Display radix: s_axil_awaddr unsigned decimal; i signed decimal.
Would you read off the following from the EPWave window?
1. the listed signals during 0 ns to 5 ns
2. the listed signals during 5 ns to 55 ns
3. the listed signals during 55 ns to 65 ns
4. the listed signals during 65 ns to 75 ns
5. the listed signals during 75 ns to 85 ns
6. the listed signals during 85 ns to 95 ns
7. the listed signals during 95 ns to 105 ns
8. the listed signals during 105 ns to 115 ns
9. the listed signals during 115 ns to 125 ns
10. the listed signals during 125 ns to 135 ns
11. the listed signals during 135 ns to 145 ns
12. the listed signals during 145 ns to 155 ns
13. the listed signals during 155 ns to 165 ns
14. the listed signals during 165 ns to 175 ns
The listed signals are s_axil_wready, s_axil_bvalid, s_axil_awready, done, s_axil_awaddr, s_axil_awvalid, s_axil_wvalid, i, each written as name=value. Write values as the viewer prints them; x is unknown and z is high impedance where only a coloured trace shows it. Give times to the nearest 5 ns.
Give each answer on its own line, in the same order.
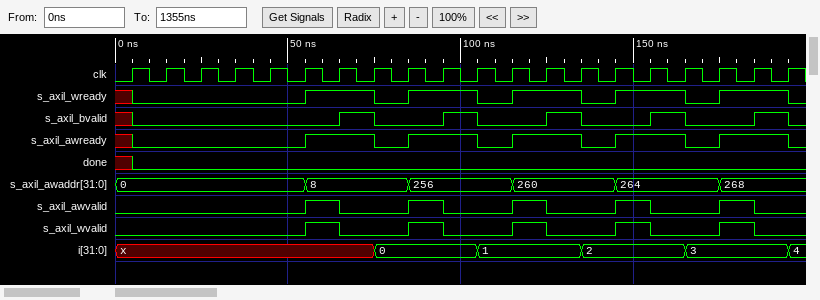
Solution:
s_axil_wready=x, s_axil_bvalid=x, s_axil_awready=x, done=x, s_axil_awaddr=0, s_axil_awvalid=0, s_axil_wvalid=0, i=x
s_axil_wready=0, s_axil_bvalid=0, s_axil_awready=0, done=0, s_axil_awaddr=0, s_axil_awvalid=0, s_axil_wvalid=0, i=x
s_axil_wready=1, s_axil_bvalid=0, s_axil_awready=1, done=0, s_axil_awaddr=8, s_axil_awvalid=1, s_axil_wvalid=1, i=x
s_axil_wready=1, s_axil_bvalid=1, s_axil_awready=1, done=0, s_axil_awaddr=8, s_axil_awvalid=0, s_axil_wvalid=0, i=x
s_axil_wready=0, s_axil_bvalid=0, s_axil_awready=0, done=0, s_axil_awaddr=8, s_axil_awvalid=0, s_axil_wvalid=0, i=0
s_axil_wready=1, s_axil_bvalid=0, s_axil_awready=1, done=0, s_axil_awaddr=256, s_axil_awvalid=1, s_axil_wvalid=1, i=0
s_axil_wready=1, s_axil_bvalid=1, s_axil_awready=1, done=0, s_axil_awaddr=256, s_axil_awvalid=0, s_axil_wvalid=0, i=0
s_axil_wready=0, s_axil_bvalid=0, s_axil_awready=0, done=0, s_axil_awaddr=256, s_axil_awvalid=0, s_axil_wvalid=0, i=1
s_axil_wready=1, s_axil_bvalid=0, s_axil_awready=1, done=0, s_axil_awaddr=260, s_axil_awvalid=1, s_axil_wvalid=1, i=1
s_axil_wready=1, s_axil_bvalid=1, s_axil_awready=1, done=0, s_axil_awaddr=260, s_axil_awvalid=0, s_axil_wvalid=0, i=1
s_axil_wready=0, s_axil_bvalid=0, s_axil_awready=0, done=0, s_axil_awaddr=260, s_axil_awvalid=0, s_axil_wvalid=0, i=2
s_axil_wready=1, s_axil_bvalid=0, s_axil_awready=1, done=0, s_axil_awaddr=264, s_axil_awvalid=1, s_axil_wvalid=1, i=2
s_axil_wready=1, s_axil_bvalid=1, s_axil_awready=1, done=0, s_axil_awaddr=264, s_axil_awvalid=0, s_axil_wvalid=0, i=2
s_axil_wready=0, s_axil_bvalid=0, s_axil_awready=0, done=0, s_axil_awaddr=264, s_axil_awvalid=0, s_axil_wvalid=0, i=3
